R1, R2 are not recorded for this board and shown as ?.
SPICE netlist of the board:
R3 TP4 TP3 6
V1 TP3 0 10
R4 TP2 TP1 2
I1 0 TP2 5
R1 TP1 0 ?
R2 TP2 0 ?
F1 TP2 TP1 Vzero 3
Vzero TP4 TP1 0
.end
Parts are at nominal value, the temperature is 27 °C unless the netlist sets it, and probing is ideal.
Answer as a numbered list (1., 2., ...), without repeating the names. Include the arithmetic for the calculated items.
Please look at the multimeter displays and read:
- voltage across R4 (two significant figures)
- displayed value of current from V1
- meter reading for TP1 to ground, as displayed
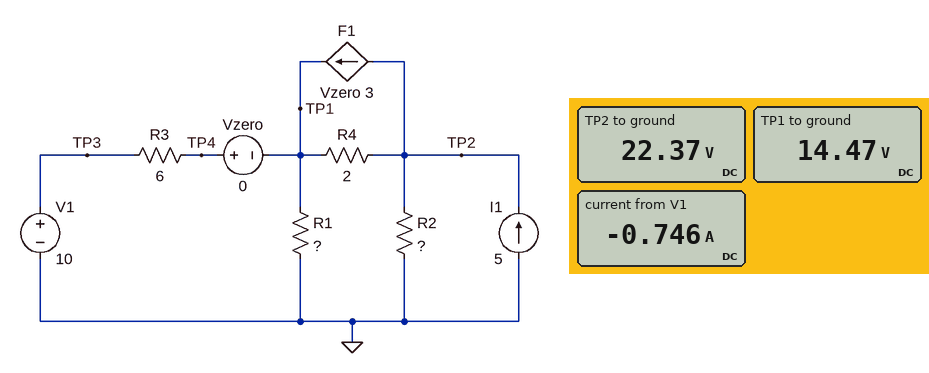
1. 22.37 V - 14.47 V = 7.9 V
2. -0.746 A
3. 14.47 V
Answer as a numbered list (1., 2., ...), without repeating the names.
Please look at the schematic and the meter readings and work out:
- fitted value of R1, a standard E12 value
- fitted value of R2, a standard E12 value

1. 15 Ω
2. 6.8 Ω
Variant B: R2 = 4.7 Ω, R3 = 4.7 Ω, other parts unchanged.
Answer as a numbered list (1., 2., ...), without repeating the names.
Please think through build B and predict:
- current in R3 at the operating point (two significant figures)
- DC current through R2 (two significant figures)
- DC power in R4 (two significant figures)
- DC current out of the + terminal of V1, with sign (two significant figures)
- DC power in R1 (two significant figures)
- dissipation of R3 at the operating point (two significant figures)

1. 460 mA
2. 3.7 A
3. 14 W
4. -460 mA
5. 9.9 W
6. 1.0 W
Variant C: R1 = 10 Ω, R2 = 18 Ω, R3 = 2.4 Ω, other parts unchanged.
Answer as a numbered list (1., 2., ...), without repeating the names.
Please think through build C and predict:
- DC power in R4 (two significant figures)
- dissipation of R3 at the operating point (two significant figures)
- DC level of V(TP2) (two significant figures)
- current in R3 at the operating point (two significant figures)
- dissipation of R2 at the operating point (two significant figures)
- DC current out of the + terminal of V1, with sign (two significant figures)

1. 150 W
2. 7.8 W
3. 32 V
4. 1.8 A
5. 56 W
6. -1.8 A
